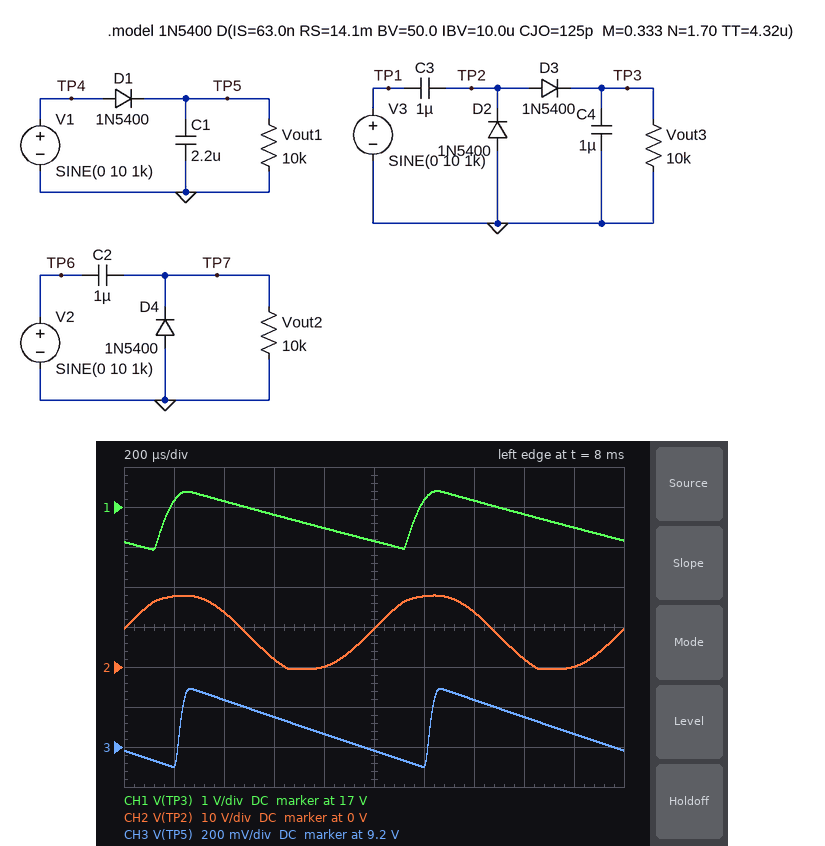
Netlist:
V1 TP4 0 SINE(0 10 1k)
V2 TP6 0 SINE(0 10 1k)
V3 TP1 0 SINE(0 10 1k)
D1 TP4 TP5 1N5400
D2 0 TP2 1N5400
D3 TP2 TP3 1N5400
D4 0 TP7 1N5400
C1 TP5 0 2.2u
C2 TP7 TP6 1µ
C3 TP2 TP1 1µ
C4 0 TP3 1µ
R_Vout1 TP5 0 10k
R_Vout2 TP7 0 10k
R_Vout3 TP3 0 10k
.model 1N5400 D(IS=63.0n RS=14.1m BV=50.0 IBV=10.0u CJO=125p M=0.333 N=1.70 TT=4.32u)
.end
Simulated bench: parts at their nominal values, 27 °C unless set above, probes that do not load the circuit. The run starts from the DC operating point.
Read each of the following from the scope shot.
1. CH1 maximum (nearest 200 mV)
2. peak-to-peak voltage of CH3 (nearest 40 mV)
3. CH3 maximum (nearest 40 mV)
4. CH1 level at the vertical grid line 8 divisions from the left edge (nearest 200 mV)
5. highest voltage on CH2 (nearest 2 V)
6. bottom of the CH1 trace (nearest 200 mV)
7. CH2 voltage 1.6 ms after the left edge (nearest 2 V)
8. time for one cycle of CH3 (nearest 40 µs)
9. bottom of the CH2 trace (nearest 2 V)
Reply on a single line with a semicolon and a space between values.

17.4 V; 400 mV; 9.48 V; 16.8 V; 18 V; 16.0 V; 2 V; 1.00 ms; 0 V
